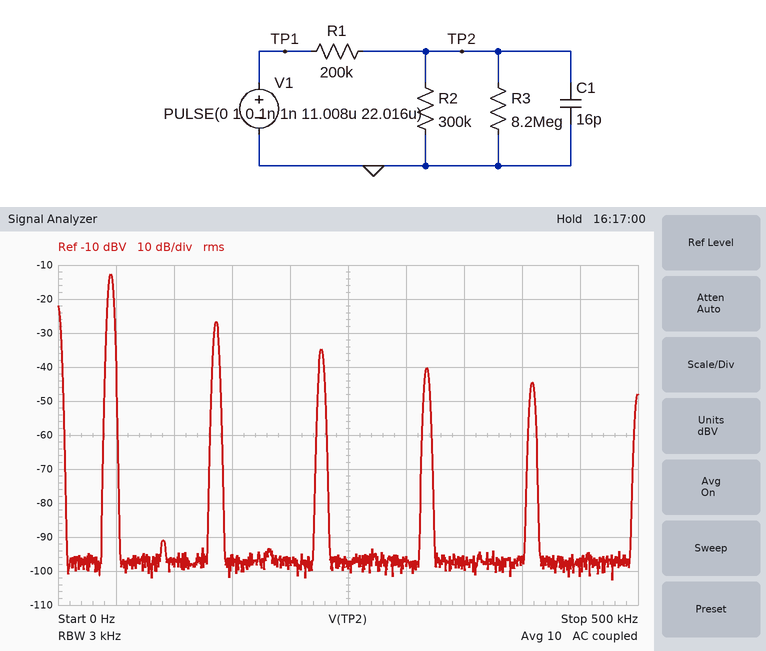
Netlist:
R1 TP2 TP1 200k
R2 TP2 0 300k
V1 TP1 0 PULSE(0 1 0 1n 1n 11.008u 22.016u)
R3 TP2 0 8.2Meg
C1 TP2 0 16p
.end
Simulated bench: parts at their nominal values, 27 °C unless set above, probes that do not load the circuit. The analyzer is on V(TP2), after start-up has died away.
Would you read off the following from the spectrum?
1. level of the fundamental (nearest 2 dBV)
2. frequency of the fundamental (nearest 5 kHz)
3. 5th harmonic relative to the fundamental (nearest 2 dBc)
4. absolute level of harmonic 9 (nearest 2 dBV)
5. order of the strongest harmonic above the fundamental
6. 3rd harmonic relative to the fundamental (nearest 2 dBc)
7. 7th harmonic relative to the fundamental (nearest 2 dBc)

-12 dBV
45 kHz
-22 dBc
-44 dBV
3
-14 dBc
-28 dBc
